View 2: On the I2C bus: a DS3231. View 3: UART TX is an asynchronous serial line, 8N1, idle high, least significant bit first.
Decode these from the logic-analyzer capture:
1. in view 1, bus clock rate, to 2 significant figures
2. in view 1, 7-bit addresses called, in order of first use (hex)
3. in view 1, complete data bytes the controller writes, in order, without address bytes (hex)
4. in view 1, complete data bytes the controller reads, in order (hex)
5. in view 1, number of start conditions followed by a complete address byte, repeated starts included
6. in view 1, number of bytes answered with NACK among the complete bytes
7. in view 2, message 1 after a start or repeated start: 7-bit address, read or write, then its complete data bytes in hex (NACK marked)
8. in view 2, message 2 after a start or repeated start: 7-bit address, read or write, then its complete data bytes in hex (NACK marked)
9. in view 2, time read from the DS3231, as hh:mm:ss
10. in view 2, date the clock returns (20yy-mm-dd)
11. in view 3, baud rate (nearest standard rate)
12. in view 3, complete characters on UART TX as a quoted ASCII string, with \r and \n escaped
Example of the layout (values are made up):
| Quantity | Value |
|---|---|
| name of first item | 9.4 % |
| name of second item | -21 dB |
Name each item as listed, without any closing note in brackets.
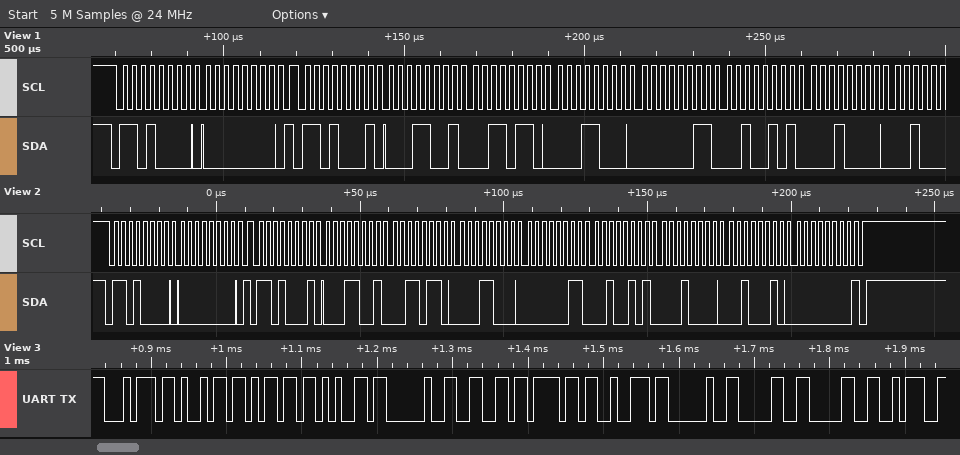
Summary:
| Quantity | Value |
|---|---|
| in view 1, bus clock rate, to 2 significant figures | 400 kHz |
| in view 1, 7-bit addresses called, in order of first use | 0x68 |
| in view 1, complete data bytes the controller writes, in order, without address bytes | 00 |
| in view 1, complete data bytes the controller reads, in order | 19 36 18 03 25 10 |
| in view 1, number of start conditions followed by a complete address byte, repeated starts included | 2 |
| in view 1, number of bytes answered with NACK among the complete bytes | 0 |
| in view 2, message 1 after a start or repeated start: 7-bit address, read or write, then its complete data bytes in hex | 0x68 write: 00 |
| in view 2, message 2 after a start or repeated start: 7-bit address, read or write, then its complete data bytes in hex | 0x68 read: 19 36 18 03 25 10 22 00 NACK |
| in view 2, time read from the DS3231, as hh:mm:ss | 18:36:19 |
| in view 2, date the clock returns | 2022-10-25 |
| in view 3, baud rate | 115200 baud |
| in view 3, complete characters on UART TX as a quoted ASCII string, with \r and \n escaped | "time for 00:" |
